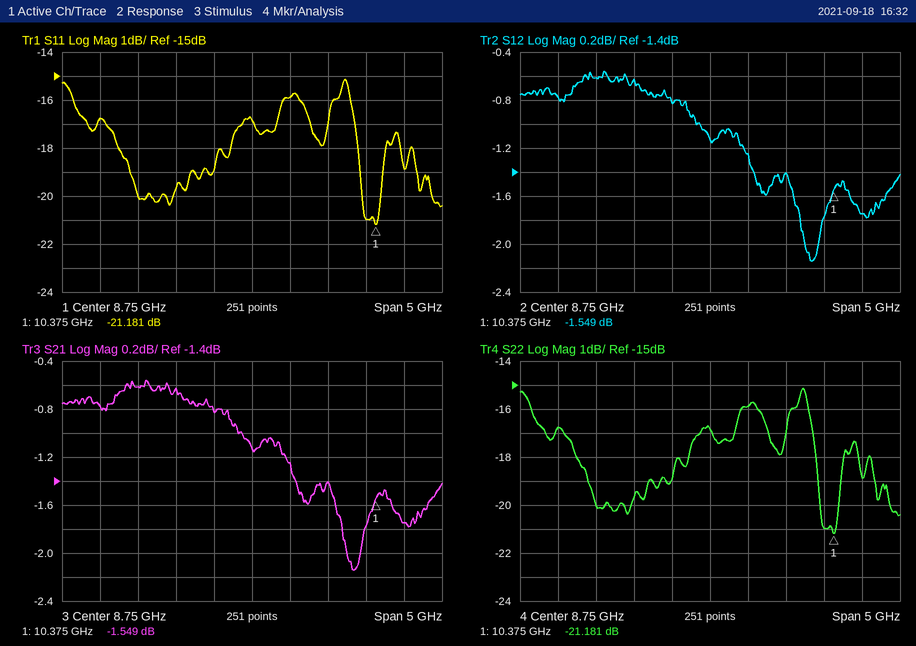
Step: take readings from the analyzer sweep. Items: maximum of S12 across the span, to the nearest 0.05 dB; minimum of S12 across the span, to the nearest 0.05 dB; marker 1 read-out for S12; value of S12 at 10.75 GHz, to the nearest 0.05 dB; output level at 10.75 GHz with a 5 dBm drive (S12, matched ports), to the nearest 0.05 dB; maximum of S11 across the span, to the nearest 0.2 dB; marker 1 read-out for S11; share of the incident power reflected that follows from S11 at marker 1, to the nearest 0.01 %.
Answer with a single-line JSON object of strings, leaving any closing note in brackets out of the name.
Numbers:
{"maximum of S12 across the span, to the nearest 0.05 dB": "-0.55 dB", "minimum of S12 across the span, to the nearest 0.05 dB": "-2.15 dB", "marker 1 read-out for S12": "-1.549 dB", "value of S12 at 10.75 GHz, to the nearest 0.05 dB": "-1.75 dB", "output level at 10.75 GHz with a 5 dBm drive (S12, matched ports), to the nearest 0.05 dB": "3.25 dBm", "maximum of S11 across the span, to the nearest 0.2 dB": "-15.2 dB", "marker 1 read-out for S11": "-21.181 dB", "share of the incident power reflected that follows from S11 at marker 1, to the nearest 0.01 %": "0.76 %"}
